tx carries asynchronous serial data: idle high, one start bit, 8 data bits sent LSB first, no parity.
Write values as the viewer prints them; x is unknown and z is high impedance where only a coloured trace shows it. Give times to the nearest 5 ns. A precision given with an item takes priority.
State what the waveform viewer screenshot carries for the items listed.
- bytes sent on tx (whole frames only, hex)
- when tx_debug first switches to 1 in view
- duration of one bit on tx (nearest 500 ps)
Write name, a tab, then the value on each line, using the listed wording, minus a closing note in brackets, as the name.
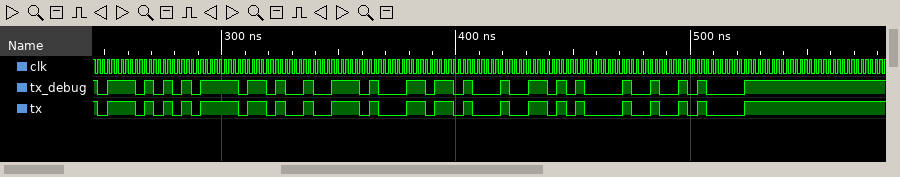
bytes sent on tx	57, 6F, 72, 6C, 64, 21, 0A
when tx_debug first switches to 1 in view	250 ns
duration of one bit on tx	4000 ps
